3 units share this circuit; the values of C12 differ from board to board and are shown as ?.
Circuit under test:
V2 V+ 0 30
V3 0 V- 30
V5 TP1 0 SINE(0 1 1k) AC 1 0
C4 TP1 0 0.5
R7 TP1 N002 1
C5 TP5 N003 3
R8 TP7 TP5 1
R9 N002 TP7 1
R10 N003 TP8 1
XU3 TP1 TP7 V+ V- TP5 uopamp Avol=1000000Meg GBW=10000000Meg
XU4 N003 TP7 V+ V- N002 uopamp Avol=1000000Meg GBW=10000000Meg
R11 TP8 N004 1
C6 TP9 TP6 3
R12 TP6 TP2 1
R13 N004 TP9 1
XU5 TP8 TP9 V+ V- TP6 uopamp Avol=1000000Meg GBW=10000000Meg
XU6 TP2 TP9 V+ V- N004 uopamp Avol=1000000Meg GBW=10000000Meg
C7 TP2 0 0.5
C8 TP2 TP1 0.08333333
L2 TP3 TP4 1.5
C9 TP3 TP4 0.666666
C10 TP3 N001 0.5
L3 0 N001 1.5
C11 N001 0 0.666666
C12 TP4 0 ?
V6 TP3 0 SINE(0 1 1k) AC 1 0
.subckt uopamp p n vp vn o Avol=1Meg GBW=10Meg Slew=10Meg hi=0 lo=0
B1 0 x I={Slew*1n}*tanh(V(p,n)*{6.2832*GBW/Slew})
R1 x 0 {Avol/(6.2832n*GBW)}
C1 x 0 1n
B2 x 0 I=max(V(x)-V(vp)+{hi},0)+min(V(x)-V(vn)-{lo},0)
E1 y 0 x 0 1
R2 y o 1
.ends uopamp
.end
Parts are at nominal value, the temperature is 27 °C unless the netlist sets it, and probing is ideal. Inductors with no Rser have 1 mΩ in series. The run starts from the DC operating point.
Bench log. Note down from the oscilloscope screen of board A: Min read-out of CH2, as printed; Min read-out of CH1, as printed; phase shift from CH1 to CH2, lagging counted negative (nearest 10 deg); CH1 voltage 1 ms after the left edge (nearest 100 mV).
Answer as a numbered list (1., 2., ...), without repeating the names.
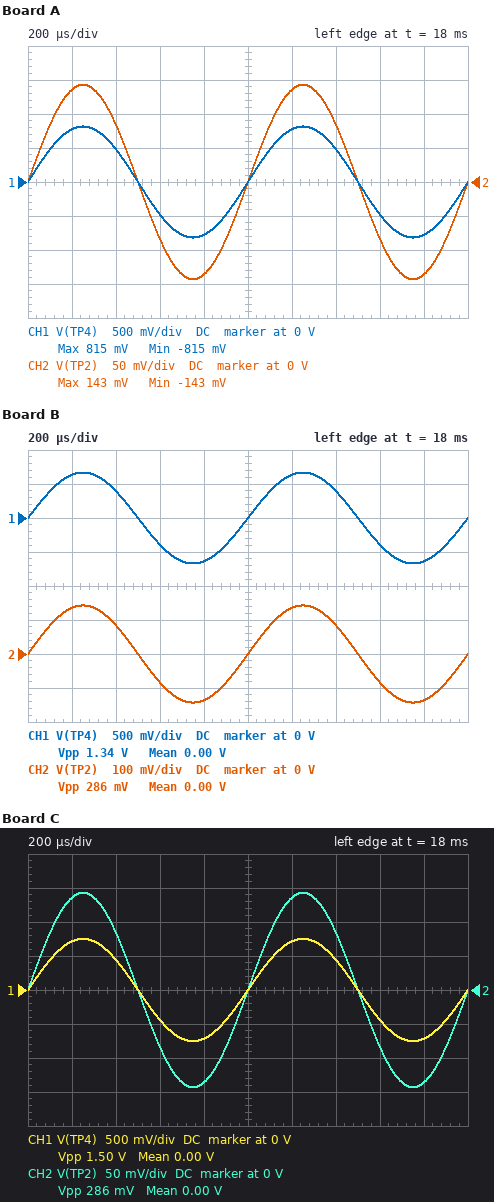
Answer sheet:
1. -143 mV
2. -815 mV
3. 0 deg
4. 0 V
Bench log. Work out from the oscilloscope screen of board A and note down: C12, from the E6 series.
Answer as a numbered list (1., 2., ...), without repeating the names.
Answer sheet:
1. 150 mF
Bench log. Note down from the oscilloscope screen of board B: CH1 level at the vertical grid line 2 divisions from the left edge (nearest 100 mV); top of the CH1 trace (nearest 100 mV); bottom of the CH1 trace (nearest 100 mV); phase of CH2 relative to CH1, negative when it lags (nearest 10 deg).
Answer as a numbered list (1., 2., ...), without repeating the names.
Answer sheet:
1. 400 mV
2. 700 mV
3. -700 mV
4. 0 deg
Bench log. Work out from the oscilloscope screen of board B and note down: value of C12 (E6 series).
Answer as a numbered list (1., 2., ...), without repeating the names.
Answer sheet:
1. 330 mF
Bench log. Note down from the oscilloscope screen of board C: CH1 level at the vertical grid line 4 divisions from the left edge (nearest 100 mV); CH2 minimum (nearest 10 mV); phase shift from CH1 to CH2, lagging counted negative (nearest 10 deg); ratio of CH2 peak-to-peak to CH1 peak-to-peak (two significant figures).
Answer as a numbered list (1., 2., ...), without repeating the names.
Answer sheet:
1. -700 mV
2. -140 mV
3. 0 deg
4. 0.19
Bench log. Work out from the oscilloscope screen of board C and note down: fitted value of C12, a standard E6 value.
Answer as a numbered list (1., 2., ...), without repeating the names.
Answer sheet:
1. 220 mF
